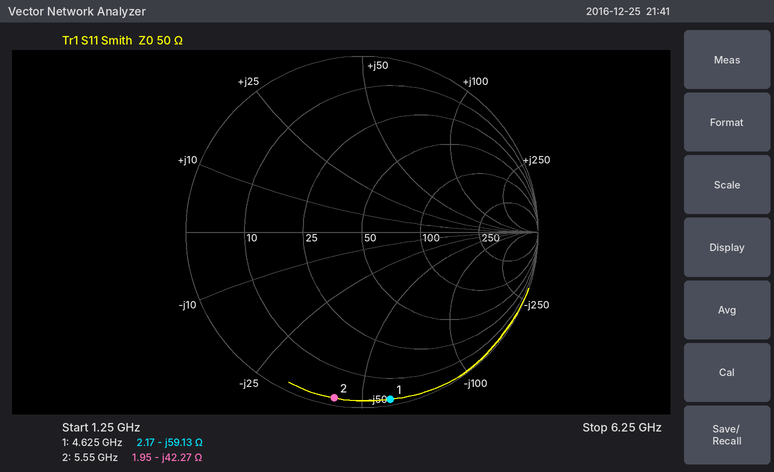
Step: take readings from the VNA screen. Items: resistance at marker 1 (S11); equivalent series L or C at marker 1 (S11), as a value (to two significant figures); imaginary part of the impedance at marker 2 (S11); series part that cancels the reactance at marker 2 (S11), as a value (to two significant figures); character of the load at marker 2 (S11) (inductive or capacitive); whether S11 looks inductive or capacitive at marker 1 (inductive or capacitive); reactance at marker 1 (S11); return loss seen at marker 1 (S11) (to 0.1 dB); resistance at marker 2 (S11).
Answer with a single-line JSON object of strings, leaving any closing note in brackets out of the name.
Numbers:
{"resistance at marker 1": "2.17 Ω", "equivalent series L or C at marker 1 (S11), as a value": "580 fF", "imaginary part of the impedance at marker 2": "-42.27 Ω", "series part that cancels the reactance at marker 2 (S11), as a value": "1.2 nH", "character of the load at marker 2 (S11)": "capacitive", "whether S11 looks inductive or capacitive at marker 1": "capacitive", "reactance at marker 1": "-59.13 Ω", "return loss seen at marker 1 (S11)": "0.3 dB", "resistance at marker 2": "1.95 Ω"}
